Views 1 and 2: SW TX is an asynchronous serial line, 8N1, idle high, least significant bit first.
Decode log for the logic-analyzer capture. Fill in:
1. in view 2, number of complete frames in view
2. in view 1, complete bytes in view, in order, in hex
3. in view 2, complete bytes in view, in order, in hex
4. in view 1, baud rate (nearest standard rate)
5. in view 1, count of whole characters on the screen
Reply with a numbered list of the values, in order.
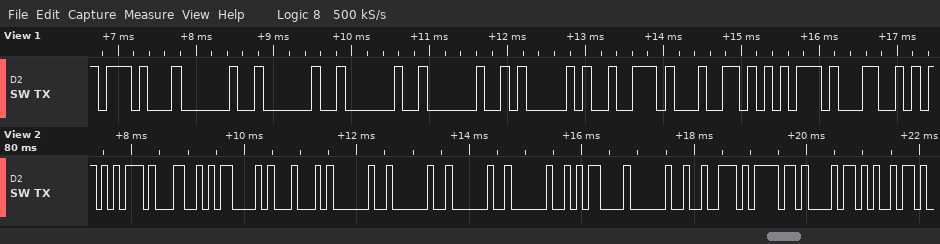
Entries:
1. 14
2. 17 20 20 20 20 41 72 64 75 4C
3. 75 4C 43 44 20 20 20 20 0D 20 72 6F 68 69
4. 9600 baud
5. 10
